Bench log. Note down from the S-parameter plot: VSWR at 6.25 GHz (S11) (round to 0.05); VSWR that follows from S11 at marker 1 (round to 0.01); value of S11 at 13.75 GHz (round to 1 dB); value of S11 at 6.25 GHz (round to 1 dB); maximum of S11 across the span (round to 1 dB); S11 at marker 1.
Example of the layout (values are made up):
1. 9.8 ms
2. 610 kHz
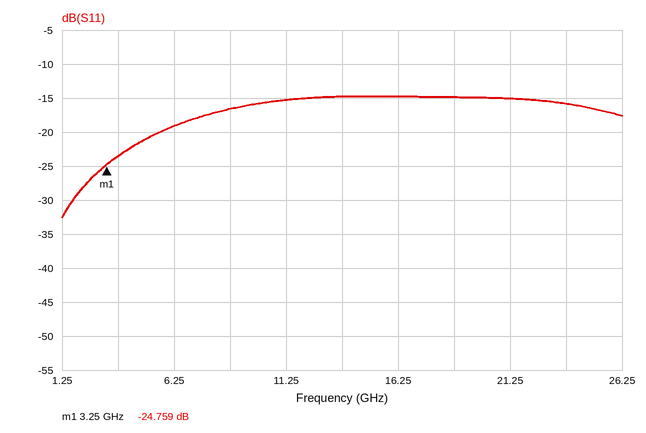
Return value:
1. 1.25
2. 1.12
3. -15 dB
4. -19 dB
5. -15 dB
6. -24.759 dB
